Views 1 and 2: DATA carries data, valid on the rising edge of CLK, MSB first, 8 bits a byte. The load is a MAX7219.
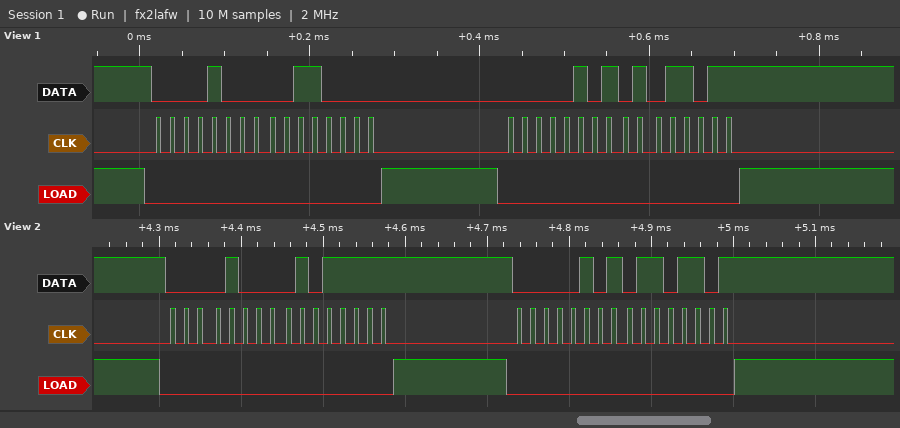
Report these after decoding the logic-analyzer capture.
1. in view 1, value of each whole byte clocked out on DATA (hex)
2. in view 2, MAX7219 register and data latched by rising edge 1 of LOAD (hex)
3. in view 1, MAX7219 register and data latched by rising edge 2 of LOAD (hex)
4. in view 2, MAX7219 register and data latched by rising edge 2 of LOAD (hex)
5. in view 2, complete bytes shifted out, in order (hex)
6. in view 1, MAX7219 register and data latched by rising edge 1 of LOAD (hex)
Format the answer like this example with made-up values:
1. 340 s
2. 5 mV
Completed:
1. 08 30 05 5B
2. register 0x8, data 0x5F
3. register 0x5, data 0x5B
4. register 0x5, data 0x6D
5. 0x08 0x5F 0x05 0x6D
6. register 0x8, data 0x30
